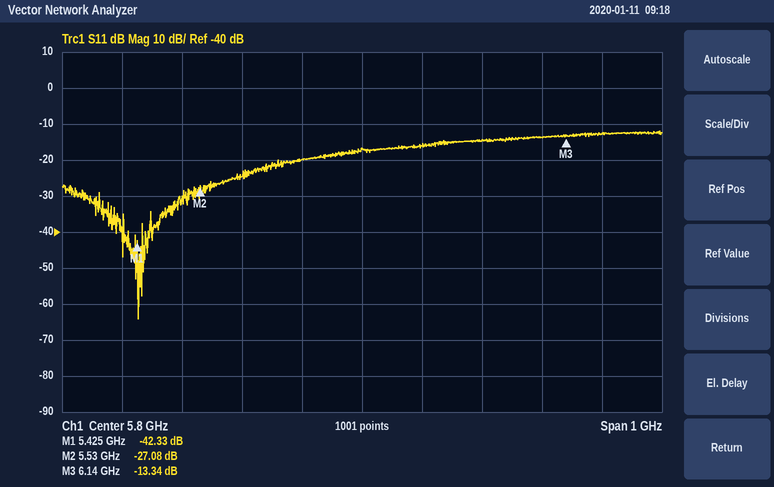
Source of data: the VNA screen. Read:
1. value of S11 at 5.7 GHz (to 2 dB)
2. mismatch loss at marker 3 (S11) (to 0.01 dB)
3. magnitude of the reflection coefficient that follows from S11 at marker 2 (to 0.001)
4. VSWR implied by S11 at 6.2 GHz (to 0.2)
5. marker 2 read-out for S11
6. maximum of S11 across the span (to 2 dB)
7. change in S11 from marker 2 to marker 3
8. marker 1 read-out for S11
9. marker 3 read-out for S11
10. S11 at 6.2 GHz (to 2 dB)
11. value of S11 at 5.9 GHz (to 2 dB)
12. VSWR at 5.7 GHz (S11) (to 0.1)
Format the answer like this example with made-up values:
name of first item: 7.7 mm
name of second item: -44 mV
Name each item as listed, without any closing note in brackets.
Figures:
value of S11 at 5.7 GHz: -20 dB
mismatch loss at marker 3 (S11): 0.21 dB
magnitude of the reflection coefficient that follows from S11 at marker 2: 0.044
VSWR implied by S11 at 6.2 GHz: 1.6
marker 2 read-out for S11: -27.08 dB
maximum of S11 across the span: -12 dB
change in S11 from marker 2 to marker 3: 13.74 dB
marker 1 read-out for S11: -42.33 dB
marker 3 read-out for S11: -13.34 dB
S11 at 6.2 GHz: -12 dB
value of S11 at 5.9 GHz: -16 dB
VSWR at 5.7 GHz (S11): 1.2
